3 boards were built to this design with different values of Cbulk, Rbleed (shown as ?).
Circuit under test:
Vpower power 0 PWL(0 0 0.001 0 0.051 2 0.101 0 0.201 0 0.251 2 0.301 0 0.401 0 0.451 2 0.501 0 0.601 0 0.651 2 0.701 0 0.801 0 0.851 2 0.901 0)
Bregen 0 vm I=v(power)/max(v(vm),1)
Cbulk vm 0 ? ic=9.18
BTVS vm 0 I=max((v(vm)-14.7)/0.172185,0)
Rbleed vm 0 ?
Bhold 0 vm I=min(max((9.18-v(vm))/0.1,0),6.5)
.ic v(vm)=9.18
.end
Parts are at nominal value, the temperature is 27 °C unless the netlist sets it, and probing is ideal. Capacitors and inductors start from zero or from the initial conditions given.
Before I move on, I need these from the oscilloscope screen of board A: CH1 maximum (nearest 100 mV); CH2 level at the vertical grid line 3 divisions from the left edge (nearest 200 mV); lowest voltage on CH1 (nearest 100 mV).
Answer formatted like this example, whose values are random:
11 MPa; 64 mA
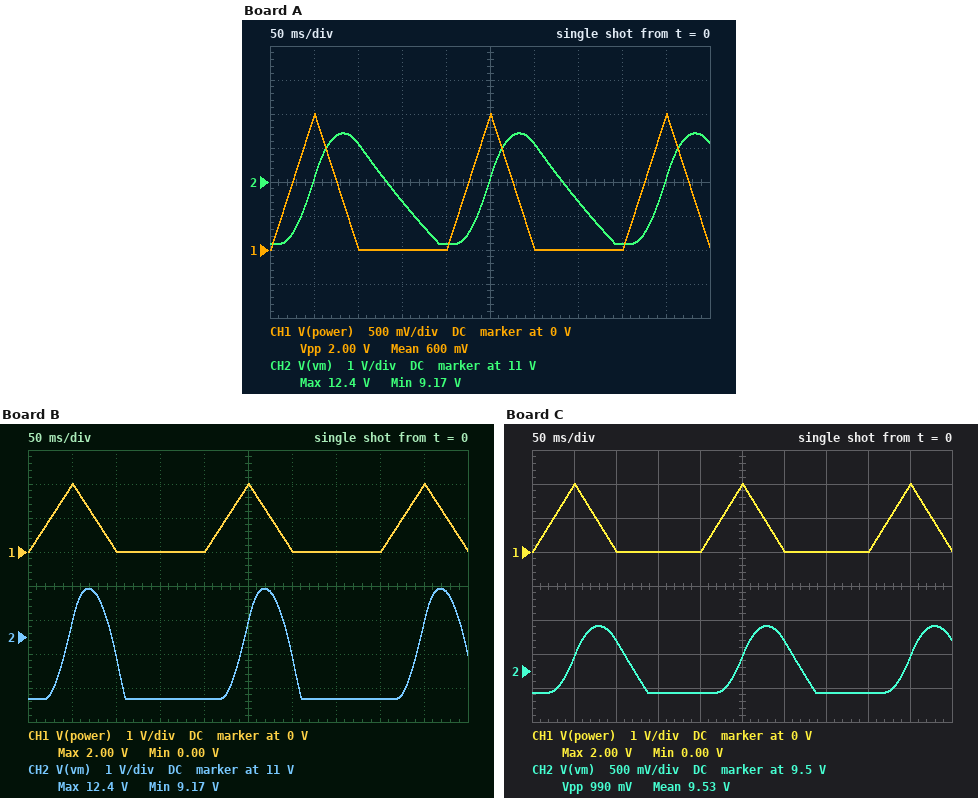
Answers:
2.0 V; 10.4 V; 0 V
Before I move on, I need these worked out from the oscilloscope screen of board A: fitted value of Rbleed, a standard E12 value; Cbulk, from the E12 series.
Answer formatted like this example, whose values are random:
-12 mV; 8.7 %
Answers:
220 Ω; 1.5 mF
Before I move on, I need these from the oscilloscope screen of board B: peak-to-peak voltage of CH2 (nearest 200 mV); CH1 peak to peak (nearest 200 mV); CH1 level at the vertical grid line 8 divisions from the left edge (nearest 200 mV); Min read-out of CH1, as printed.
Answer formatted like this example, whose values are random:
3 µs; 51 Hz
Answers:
3.2 V; 2.0 V; 0 V; 0.00 V
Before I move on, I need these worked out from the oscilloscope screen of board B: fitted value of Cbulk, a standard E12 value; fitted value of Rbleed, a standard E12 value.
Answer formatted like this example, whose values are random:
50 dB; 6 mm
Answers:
680 µF; 120 Ω
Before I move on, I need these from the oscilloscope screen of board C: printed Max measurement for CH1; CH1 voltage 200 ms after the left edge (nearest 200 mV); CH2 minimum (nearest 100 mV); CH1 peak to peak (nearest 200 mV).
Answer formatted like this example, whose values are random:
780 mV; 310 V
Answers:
2.00 V; 0 V; 9.2 V; 2.0 V
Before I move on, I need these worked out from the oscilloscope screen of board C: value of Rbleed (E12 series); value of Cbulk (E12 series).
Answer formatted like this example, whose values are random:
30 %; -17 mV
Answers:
120 Ω; 3.9 mF
